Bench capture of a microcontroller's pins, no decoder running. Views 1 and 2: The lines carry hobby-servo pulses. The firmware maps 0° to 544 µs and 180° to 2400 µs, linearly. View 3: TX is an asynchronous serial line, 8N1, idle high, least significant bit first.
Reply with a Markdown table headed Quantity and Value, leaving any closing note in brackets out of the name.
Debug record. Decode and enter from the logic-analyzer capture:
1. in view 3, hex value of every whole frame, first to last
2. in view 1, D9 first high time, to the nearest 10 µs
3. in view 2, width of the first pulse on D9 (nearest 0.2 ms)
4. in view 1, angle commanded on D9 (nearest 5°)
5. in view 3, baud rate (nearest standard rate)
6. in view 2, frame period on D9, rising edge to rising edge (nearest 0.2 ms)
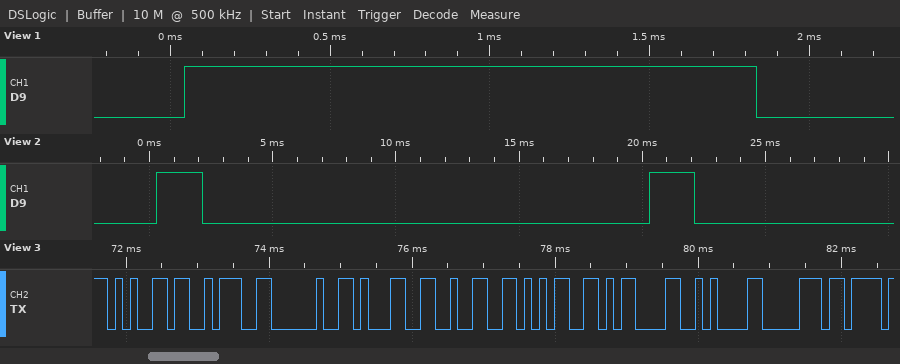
| Quantity | Value |
|---|---|
| in view 3, hex value of every whole frame, first to last | 0x65 0x3A 0x20 0x31 0x32 0x35 0x0D 0x0A 0x70 |
| in view 1, D9 first high time, to the nearest 10 µs | 1790 µs |
| in view 2, width of the first pulse on D9 | 1.8 ms |
| in view 1, angle commanded on D9 | 120° |
| in view 3, baud rate | 9600 baud |
| in view 2, frame period on D9, rising edge to rising edge | 20.0 ms |
